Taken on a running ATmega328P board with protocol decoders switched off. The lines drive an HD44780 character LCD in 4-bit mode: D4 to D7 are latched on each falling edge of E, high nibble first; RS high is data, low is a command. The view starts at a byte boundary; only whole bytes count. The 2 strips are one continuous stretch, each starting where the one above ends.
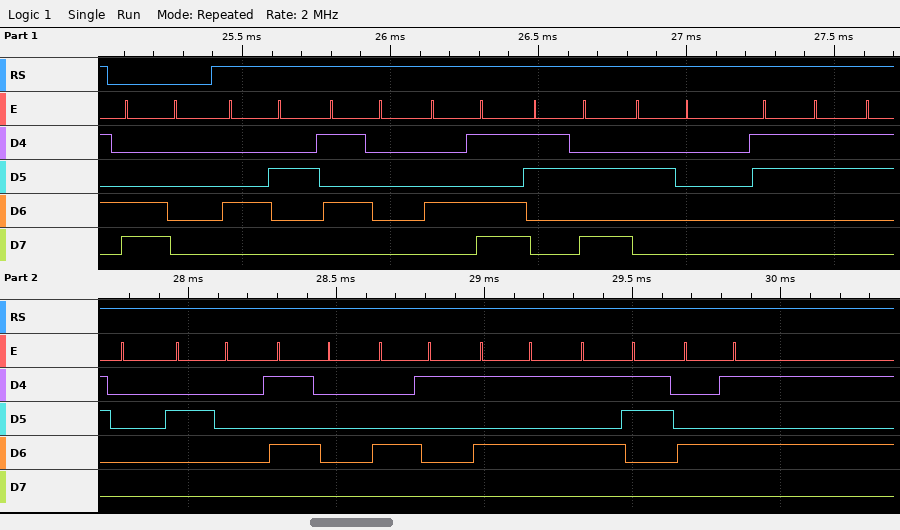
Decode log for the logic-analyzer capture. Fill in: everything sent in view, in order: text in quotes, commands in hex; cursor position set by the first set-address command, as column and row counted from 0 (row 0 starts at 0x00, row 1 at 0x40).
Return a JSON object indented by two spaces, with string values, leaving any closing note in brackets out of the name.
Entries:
{
  "everything sent in view, in order: text in quotes, commands in hex": "0xC0 \"BPM: 30 PAUSE\"",
  "cursor position set by the first set-address command, as column and row counted from 0": "column 0, row 1"
}
